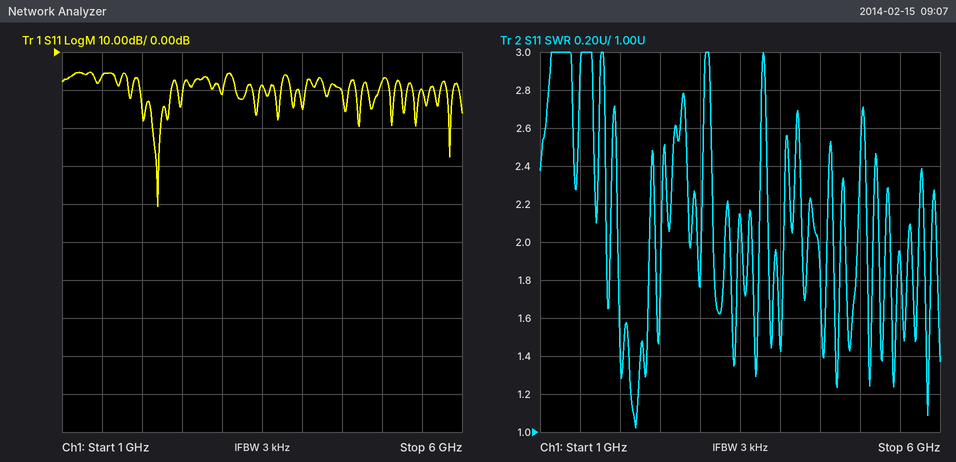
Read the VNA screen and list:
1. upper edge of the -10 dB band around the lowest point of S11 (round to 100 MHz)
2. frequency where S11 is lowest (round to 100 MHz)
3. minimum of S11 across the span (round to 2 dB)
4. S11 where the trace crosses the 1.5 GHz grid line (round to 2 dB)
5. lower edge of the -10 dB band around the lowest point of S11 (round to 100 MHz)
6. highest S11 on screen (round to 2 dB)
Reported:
2.4 GHz
2.2 GHz
-40 dB
-6 dB
2.0 GHz
-6 dB
